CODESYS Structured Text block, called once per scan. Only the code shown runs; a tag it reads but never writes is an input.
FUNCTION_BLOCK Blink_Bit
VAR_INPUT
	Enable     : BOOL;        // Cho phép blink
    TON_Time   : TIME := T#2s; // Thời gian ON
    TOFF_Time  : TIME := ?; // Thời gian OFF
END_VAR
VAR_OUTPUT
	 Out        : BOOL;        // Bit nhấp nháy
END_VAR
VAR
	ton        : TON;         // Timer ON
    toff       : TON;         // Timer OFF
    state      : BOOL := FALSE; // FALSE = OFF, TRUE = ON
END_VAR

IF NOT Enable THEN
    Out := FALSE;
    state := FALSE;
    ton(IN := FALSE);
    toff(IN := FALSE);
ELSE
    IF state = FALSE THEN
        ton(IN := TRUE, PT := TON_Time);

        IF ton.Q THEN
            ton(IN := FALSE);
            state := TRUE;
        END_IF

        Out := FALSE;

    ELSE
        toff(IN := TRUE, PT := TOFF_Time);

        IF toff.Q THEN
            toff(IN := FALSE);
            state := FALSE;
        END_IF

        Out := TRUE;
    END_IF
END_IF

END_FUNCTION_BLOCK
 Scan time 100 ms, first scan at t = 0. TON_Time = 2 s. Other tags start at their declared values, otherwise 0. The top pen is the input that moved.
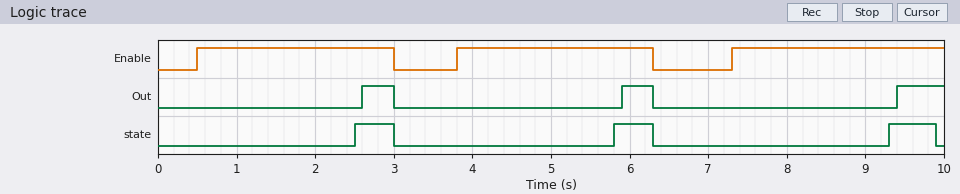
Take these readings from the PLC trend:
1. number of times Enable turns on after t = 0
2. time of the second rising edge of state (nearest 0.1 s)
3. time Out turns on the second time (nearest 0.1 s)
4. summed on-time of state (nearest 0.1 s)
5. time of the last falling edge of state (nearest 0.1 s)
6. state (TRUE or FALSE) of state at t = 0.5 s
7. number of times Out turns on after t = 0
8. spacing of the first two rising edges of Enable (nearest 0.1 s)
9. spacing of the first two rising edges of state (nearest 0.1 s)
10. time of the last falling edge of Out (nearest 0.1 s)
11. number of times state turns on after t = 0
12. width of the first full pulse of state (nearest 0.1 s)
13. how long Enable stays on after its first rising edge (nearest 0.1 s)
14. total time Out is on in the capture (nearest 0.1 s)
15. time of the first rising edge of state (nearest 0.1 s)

3
5.8 s
5.9 s
1.6 s
9.9 s
FALSE
3
3.3 s
3.3 s
6.3 s
3
0.5 s
2.5 s
1.4 s
2.5 s
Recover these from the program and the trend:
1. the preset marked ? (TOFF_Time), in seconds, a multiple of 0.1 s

0.5 s
